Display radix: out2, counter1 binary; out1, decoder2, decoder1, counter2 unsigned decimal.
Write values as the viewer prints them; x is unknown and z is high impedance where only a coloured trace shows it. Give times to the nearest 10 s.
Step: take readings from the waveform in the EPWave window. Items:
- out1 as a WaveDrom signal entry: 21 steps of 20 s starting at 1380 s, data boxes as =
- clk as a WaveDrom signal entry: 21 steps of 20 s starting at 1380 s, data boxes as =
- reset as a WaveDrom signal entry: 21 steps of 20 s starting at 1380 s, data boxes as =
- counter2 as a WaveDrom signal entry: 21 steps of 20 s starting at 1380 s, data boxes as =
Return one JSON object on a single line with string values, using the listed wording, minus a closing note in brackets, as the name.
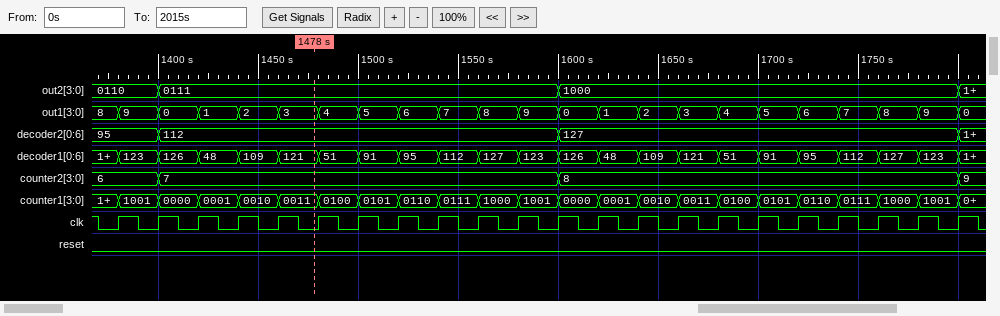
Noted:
{"out1 as a WaveDrom signal entry: 21 steps of 20 s starting at 1380 s, data boxes as =": "{name: 'out1', wave: '=====================', data: '9 0 1 2 3 4 5 6 7 8 9 0 1 2 3 4 5 6 7 8 9'}", "clk as a WaveDrom signal entry: 21 steps of 20 s starting at 1380 s, data boxes as =": "{name: 'clk', wave: 'p....................'}", "reset as a WaveDrom signal entry: 21 steps of 20 s starting at 1380 s, data boxes as =": "{name: 'reset', wave: '0....................'}", "counter2 as a WaveDrom signal entry: 21 steps of 20 s starting at 1380 s, data boxes as =": "{name: 'counter2', wave: '==.........=.........', data: '6 7 8'}"}
